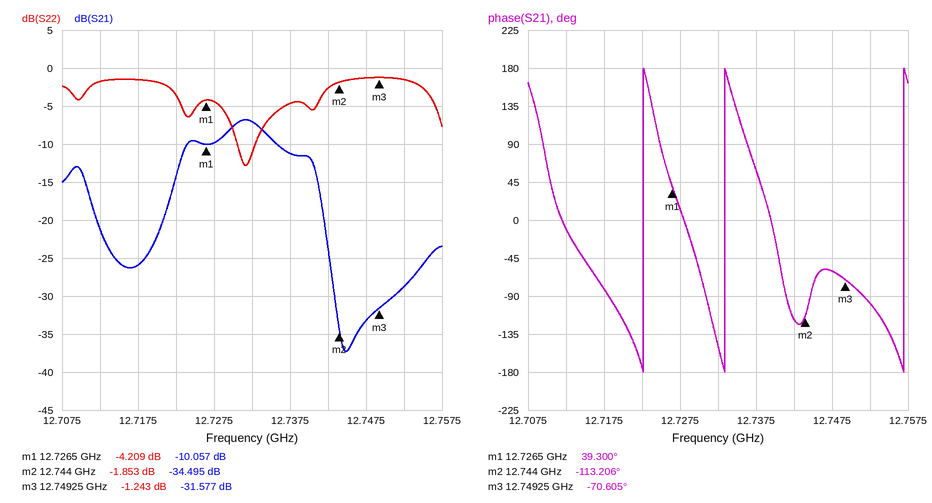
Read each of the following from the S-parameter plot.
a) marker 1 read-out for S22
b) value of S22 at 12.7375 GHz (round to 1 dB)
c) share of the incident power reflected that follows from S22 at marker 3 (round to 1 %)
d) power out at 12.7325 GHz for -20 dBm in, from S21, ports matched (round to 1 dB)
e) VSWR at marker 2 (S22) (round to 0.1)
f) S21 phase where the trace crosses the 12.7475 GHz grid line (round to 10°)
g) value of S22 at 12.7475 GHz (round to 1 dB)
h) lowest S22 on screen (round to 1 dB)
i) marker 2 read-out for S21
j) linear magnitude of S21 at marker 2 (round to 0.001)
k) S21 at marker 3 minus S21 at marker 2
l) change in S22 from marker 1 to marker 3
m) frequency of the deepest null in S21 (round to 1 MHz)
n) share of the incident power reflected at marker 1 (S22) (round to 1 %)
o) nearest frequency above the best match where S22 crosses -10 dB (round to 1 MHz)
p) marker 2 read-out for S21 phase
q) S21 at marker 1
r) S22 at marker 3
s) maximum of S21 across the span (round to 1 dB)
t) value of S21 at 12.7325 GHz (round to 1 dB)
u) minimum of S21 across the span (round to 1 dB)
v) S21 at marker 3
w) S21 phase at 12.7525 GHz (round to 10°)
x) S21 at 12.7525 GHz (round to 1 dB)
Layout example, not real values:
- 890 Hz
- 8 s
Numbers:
- -4.209 dB
- -5 dB
- 75 %
- -27 dBm
- 9.4
- -60°
- -1 dB
- -13 dB
- -34.495 dB
- 0.019
- 2.918 dB
- 2.966 dB
- 12.745 GHz
- 38 %
- 12.733 GHz
- -113.206°
- -10.057 dB
- -1.243 dB
- -7 dB
- -7 dB
- -37 dB
- -31.577 dB
- -100°
- -29 dB
